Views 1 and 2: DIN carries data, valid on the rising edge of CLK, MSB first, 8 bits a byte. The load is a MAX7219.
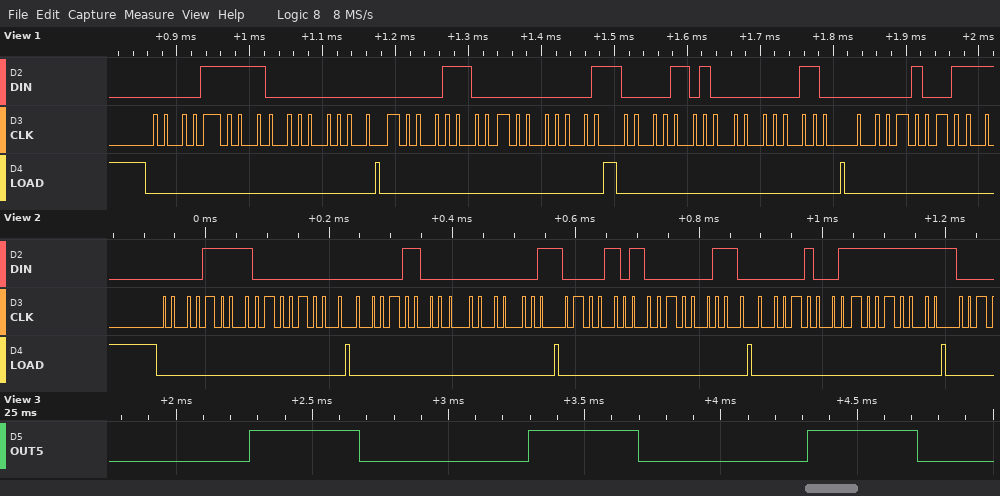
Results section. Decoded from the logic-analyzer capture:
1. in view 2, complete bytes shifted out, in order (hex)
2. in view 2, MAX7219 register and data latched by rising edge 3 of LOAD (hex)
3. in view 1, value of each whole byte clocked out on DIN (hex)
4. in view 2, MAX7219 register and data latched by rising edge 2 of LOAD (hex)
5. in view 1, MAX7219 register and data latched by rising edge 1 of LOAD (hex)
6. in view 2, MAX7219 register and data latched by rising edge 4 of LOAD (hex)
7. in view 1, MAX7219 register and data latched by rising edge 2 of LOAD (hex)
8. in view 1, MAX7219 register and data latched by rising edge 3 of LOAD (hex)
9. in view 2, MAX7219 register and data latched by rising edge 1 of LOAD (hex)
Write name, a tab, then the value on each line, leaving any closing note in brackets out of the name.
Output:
in view 2, complete bytes shifted out, in order	0x0F 0x00 0x0C 0x01 0x0A 0x06 0x09 0xFF
in view 2, MAX7219 register and data latched by rising edge 3 of LOAD	register 0xA, data 0x06
in view 1, value of each whole byte clocked out on DIN	0F 00 0C 01 0A 06 09
in view 2, MAX7219 register and data latched by rising edge 2 of LOAD	register 0xC, data 0x01
in view 1, MAX7219 register and data latched by rising edge 1 of LOAD	register 0xF, data 0x00
in view 2, MAX7219 register and data latched by rising edge 4 of LOAD	register 0x9, data 0xFF
in view 1, MAX7219 register and data latched by rising edge 2 of LOAD	register 0xC, data 0x01
in view 1, MAX7219 register and data latched by rising edge 3 of LOAD	register 0xA, data 0x06
in view 2, MAX7219 register and data latched by rising edge 1 of LOAD	register 0xF, data 0x00
